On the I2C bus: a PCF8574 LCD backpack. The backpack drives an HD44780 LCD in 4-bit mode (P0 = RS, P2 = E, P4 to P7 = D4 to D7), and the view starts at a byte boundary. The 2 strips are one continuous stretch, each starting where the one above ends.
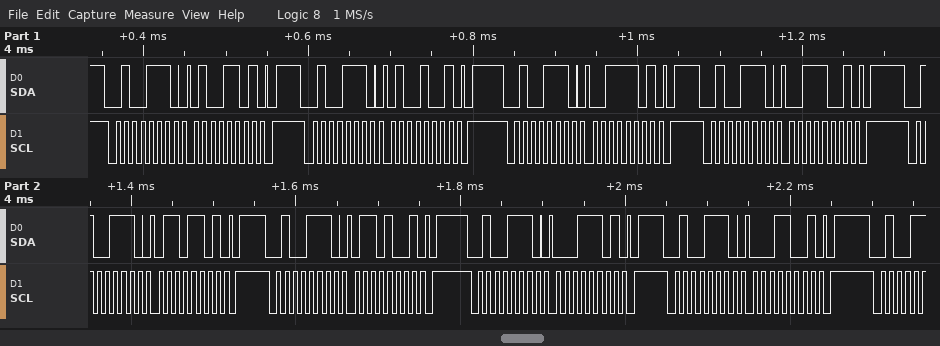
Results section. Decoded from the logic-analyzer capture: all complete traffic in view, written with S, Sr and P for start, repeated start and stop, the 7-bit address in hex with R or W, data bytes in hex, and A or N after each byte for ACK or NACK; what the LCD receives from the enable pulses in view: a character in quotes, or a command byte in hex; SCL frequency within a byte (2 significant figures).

S 27W A 4D A P S 27W A 49 A P S 27W A 3D A P S 27W A 39 A P S 27W A 6D A P S 27W A 69 A P S 27W A 1D A P S 27W A 19 A P
'C' 'a'
100 kHz
